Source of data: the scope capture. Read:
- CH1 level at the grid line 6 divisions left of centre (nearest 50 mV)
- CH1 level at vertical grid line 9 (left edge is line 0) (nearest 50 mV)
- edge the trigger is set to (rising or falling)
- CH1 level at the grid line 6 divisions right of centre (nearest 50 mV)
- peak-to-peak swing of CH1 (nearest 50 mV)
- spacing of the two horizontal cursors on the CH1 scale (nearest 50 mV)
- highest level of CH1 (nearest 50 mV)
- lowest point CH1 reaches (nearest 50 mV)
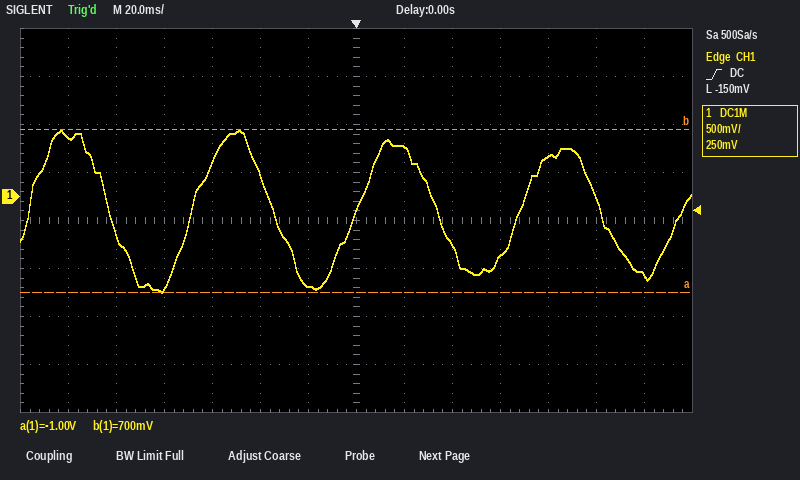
600 mV
-500 mV
rising
-800 mV
1.70 V
1.70 V
700 mV
-1.00 V
